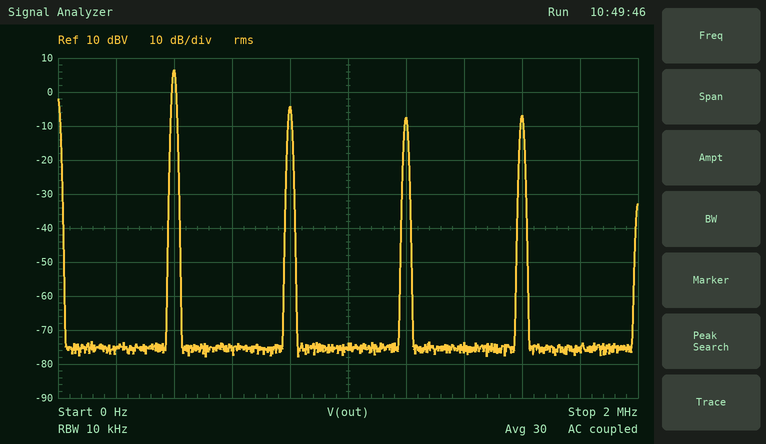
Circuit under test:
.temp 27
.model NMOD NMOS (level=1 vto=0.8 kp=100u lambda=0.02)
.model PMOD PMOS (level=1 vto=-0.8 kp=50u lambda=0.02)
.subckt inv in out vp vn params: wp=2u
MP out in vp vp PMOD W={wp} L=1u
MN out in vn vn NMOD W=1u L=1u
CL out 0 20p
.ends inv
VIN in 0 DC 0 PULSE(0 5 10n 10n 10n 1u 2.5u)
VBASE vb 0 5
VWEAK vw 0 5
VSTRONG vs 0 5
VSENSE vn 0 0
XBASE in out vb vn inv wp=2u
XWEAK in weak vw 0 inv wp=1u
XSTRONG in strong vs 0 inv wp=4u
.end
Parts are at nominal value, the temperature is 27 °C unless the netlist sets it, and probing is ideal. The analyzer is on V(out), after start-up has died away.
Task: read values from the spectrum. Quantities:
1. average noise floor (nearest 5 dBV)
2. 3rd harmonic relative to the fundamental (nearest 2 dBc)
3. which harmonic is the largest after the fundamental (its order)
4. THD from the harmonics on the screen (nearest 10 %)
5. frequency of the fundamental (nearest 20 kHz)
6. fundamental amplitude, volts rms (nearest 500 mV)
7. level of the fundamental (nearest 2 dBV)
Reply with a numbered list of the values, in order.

1. -75 dBV
2. -14 dBc
3. 2
4. 40 %
5. 400 kHz
6. 2.0 V
7. 6 dBV
